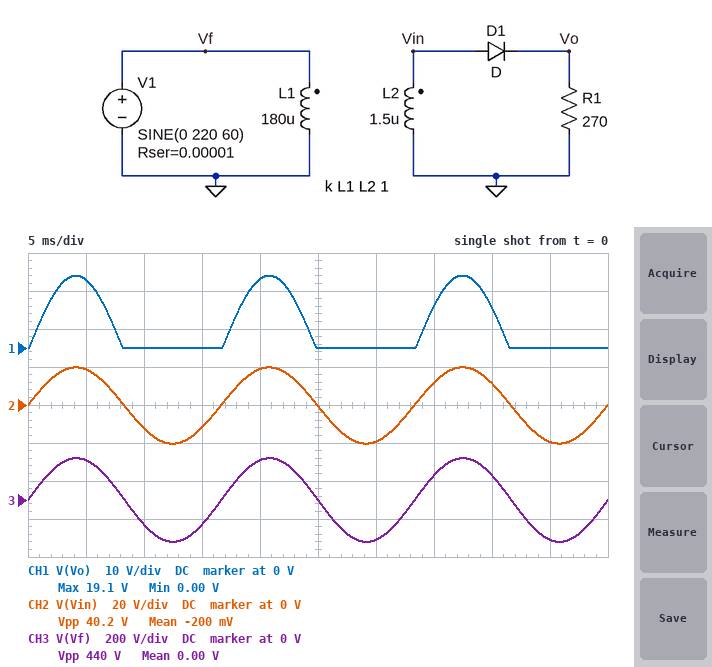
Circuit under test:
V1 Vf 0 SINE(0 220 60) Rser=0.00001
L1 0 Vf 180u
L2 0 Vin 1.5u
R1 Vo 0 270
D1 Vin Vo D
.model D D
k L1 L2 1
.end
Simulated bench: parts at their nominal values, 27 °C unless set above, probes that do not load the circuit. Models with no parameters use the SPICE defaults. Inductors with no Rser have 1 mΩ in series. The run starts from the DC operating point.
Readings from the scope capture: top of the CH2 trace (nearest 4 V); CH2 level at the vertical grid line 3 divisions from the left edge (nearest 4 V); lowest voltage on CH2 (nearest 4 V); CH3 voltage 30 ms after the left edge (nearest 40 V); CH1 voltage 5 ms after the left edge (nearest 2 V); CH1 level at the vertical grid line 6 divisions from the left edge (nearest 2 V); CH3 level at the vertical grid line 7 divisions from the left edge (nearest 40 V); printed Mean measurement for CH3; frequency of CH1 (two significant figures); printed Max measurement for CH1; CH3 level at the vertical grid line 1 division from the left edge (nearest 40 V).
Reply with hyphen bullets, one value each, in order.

- 20 V
- -12 V
- -20 V
- -200 V
- 18 V
- 0 V
- 120 V
- 0.00 V
- 60 Hz
- 19.1 V
- 200 V
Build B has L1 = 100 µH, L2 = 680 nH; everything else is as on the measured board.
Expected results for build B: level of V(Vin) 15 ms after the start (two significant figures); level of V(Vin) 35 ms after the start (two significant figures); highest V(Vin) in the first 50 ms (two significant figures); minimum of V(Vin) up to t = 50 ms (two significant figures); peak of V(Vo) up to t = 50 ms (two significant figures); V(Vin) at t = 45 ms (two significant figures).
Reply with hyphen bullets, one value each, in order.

- -11 V
- 11 V
- 18 V
- -19 V
- 17 V
- -18 V
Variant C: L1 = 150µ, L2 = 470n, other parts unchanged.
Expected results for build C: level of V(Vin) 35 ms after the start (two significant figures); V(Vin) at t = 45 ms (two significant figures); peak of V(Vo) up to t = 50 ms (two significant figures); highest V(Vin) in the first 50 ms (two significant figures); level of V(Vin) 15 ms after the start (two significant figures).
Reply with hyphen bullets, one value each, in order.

- 7.2 V
- -12 V
- 11 V
- 12 V
- -7.3 V
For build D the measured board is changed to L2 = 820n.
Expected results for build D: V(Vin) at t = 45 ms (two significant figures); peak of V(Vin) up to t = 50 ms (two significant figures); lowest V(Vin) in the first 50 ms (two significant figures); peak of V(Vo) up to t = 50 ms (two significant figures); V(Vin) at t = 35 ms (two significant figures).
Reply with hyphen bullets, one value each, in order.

- -14 V
- 15 V
- -15 V
- 14 V
- 8.7 V
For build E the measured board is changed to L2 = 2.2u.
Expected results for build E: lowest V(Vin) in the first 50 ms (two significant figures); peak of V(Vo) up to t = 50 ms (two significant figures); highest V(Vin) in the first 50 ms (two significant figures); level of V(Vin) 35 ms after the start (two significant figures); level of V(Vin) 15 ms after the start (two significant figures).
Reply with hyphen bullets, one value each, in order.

- -25 V
- 23 V
- 24 V
- 14 V
- -14 V
